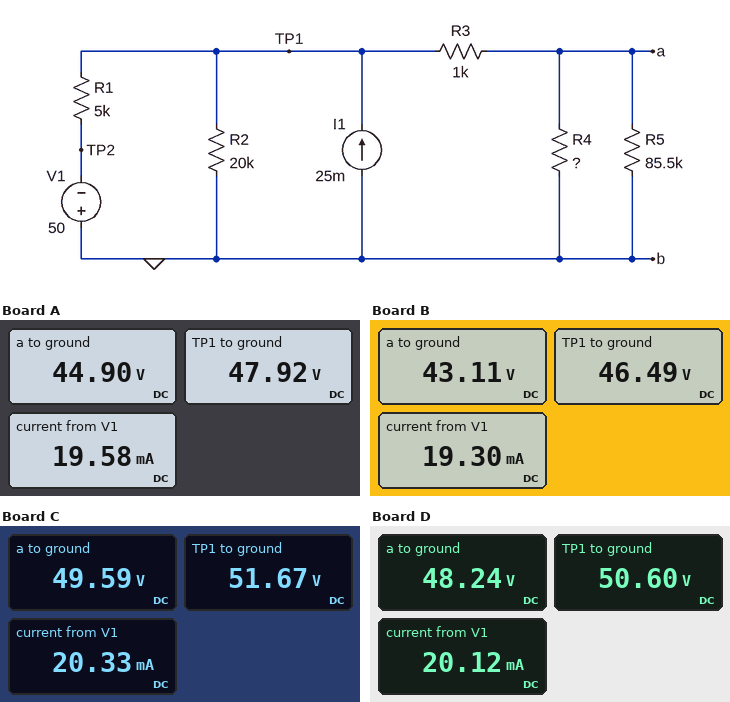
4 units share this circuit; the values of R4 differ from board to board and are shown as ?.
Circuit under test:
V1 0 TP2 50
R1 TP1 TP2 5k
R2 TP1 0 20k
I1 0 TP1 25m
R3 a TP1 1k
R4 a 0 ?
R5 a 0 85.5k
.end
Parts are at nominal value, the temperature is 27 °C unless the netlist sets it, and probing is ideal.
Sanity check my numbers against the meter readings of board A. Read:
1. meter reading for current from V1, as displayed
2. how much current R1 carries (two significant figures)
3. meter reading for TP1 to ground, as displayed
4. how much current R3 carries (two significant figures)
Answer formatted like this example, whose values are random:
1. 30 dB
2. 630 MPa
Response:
1. 19.58 mA
2. 20 mA
3. 47.92 V
4. 3.0 mA
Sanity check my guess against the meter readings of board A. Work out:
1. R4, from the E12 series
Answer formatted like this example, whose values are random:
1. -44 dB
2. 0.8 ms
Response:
1. 18 kΩ
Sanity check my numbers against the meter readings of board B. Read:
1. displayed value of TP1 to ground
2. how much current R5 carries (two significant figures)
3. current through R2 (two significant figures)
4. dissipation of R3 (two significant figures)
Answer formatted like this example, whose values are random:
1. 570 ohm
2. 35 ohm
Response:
1. 46.49 V
2. 500 µA
3. 2.3 mA
4. 11 mW
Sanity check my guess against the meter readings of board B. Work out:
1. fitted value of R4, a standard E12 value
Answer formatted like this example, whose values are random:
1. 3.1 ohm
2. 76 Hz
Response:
1. 15 kΩ
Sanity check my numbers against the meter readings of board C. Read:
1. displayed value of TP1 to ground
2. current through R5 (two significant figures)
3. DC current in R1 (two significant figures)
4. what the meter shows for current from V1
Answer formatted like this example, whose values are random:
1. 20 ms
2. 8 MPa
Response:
1. 51.67 V
2. 580 µA
3. 20 mA
4. 20.33 mA
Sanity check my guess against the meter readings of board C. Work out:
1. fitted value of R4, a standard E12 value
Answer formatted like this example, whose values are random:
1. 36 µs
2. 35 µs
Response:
1. 33 kΩ
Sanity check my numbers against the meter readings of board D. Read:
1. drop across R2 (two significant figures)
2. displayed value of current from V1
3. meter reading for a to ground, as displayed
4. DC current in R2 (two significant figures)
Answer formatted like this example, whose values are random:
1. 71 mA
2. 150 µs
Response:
1. 51 V
2. 20.12 mA
3. 48.24 V
4. 2.5 mA
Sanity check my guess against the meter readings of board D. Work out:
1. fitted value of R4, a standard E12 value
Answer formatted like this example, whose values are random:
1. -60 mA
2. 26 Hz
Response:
1. 27 kΩ
